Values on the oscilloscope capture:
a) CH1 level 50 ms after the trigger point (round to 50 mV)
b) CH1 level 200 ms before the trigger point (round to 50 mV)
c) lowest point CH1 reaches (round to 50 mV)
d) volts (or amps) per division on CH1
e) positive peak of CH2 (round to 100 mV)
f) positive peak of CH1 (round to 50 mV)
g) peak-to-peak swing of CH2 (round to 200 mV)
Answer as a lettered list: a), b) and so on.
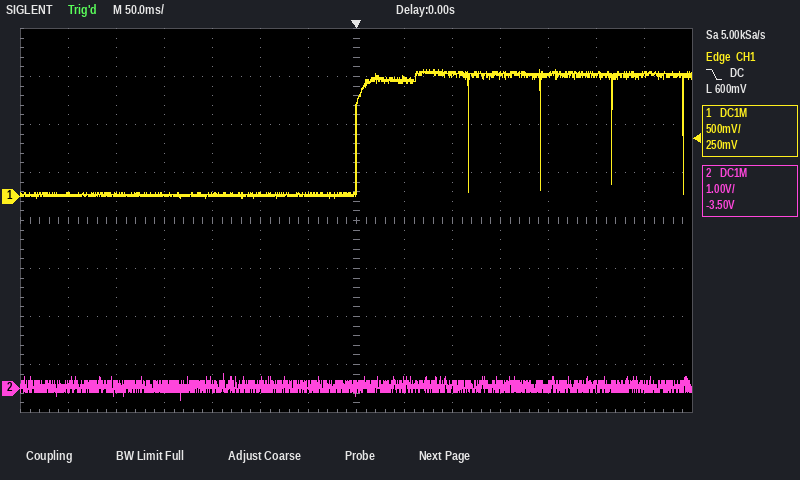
a) 1.20 V
b) 0 mV
c) 0 mV
d) 500 mV
e) 300 mV
f) 1.30 V
g) 600 mV
